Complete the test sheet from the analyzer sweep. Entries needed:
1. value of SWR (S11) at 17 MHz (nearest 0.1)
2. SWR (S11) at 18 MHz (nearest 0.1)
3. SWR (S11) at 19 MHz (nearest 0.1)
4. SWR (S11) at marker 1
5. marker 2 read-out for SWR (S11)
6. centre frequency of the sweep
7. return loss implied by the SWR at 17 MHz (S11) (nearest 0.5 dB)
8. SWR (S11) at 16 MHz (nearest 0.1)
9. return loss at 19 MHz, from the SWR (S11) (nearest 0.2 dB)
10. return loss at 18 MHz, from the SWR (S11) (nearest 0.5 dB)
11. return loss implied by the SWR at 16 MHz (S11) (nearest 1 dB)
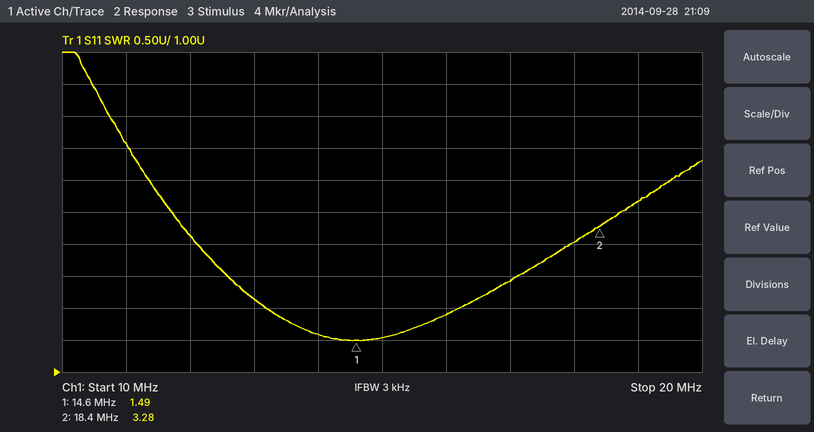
2.4
3.0
3.7
1.49
3.28
15 MHz
7.5 dB
1.9
4.8 dB
6.0 dB
10 dB
